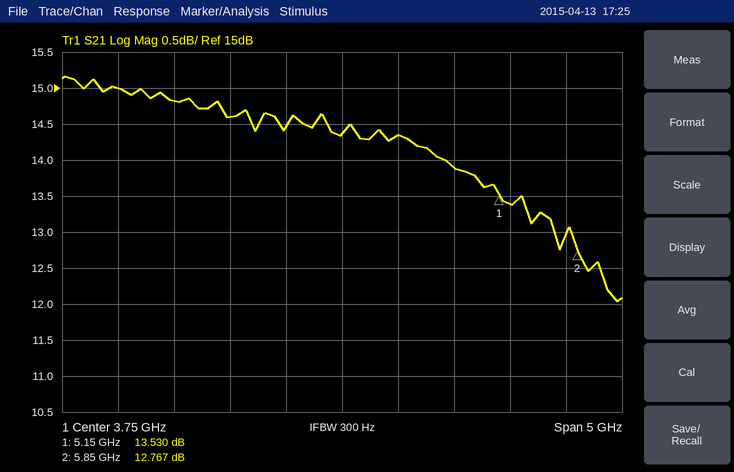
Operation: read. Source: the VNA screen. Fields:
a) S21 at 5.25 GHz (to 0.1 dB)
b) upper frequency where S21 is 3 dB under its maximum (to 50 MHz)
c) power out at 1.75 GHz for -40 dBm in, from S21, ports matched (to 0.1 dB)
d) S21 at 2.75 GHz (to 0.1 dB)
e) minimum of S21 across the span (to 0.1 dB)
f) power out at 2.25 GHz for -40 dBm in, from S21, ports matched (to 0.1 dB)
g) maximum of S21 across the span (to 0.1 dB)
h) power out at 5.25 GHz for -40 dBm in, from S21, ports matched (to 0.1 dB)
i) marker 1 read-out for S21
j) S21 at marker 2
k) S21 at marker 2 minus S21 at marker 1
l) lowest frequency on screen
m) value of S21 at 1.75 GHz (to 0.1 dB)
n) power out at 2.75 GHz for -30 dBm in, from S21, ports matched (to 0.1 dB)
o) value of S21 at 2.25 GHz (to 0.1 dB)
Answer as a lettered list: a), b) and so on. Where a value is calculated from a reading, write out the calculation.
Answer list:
a) 13.4 dB
b) 6.15 GHz
c) -40 dBm + (15.0 dB) = -25.0 dBm
d) 14.6 dB
e) 12.0 dB
f) -40 dBm + (14.8 dB) = -25.2 dBm
g) 15.2 dB
h) -40 dBm + (13.4 dB) = -26.6 dBm
i) 13.530 dB
j) 12.767 dB
k) 12.767 − (13.53) = -0.763 dB
l) 1.25 GHz
m) 15.0 dB
n) -30 dBm + (14.6 dB) = -15.4 dBm
o) 14.8 dB
